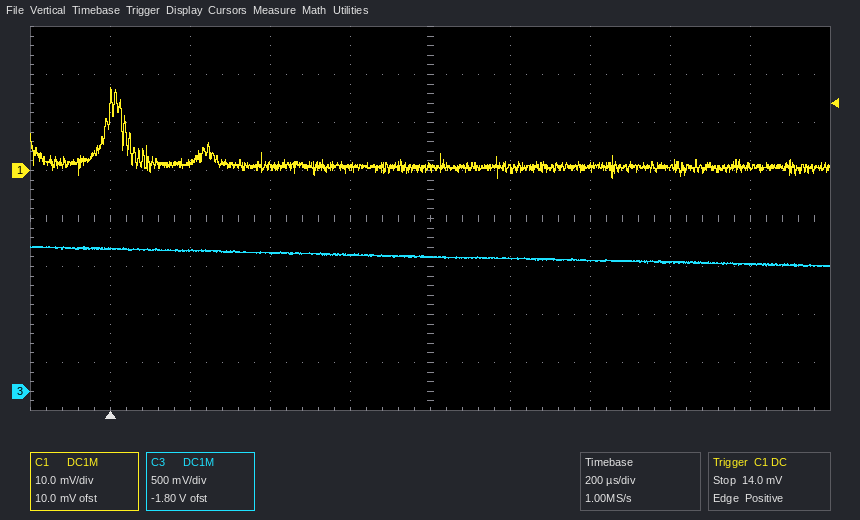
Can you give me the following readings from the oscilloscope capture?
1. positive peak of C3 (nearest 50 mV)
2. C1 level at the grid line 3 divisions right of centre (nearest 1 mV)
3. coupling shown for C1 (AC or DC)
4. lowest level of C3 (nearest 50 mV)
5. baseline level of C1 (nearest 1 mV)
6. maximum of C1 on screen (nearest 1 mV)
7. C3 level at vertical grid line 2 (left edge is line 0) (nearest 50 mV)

1.50 V
1 mV
DC
1.30 V
1 mV
17 mV
1.45 V
